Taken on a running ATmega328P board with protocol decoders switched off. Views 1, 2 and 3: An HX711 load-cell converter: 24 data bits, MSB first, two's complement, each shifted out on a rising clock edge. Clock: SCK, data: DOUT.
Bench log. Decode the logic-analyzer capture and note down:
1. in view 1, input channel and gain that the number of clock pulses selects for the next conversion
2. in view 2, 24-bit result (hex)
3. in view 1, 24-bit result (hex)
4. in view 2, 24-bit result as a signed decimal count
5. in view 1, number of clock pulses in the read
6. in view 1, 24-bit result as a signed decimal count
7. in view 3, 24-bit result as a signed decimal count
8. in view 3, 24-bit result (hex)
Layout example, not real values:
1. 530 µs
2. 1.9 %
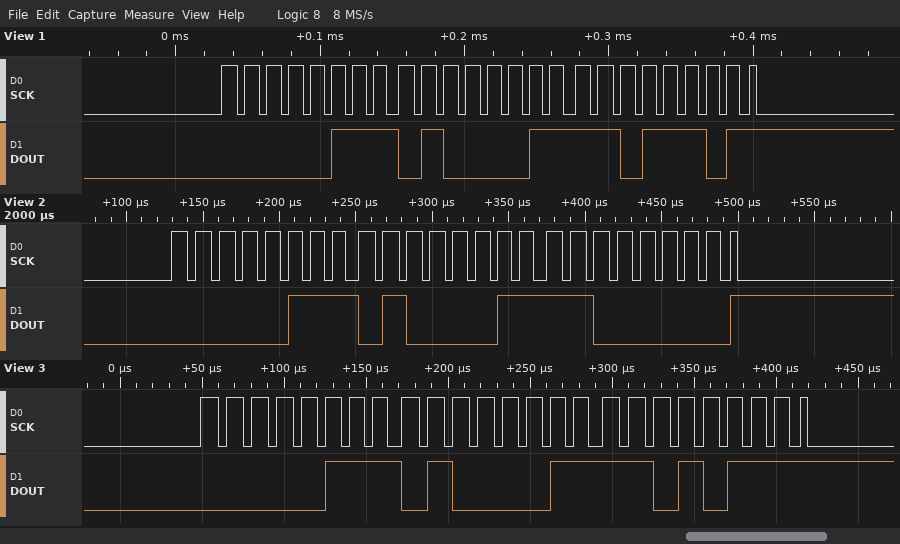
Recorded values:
1. channel A, gain 128
2. 0x0743C0
3. 0x0743DD
4. 476096
5. 25
6. 476125
7. 476119
8. 0x0743D7
